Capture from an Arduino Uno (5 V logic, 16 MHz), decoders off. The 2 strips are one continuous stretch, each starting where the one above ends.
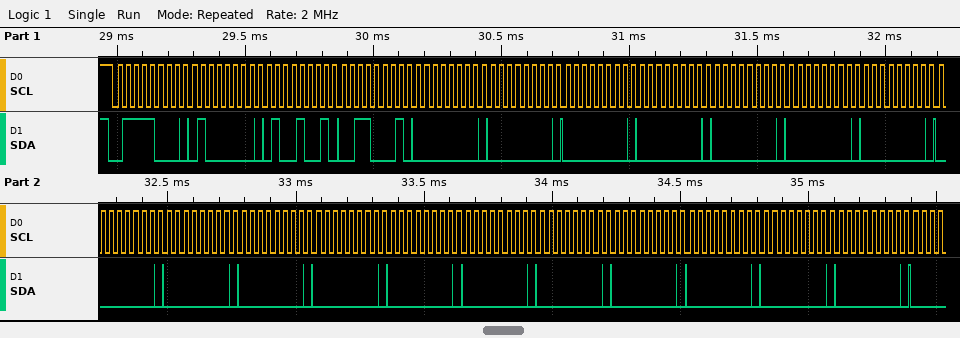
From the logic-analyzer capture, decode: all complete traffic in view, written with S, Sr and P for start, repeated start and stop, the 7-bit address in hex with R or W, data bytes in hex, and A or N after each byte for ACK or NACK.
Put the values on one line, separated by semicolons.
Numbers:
S 3CW A 40 A 49 A 31 A 00 A 00 A 00 A 00 A 00 A 00 A 00 A 00 A 00 A 00 A 00 A 00 A 00 A 00 A 00 A 00 A 00 A 00 A
